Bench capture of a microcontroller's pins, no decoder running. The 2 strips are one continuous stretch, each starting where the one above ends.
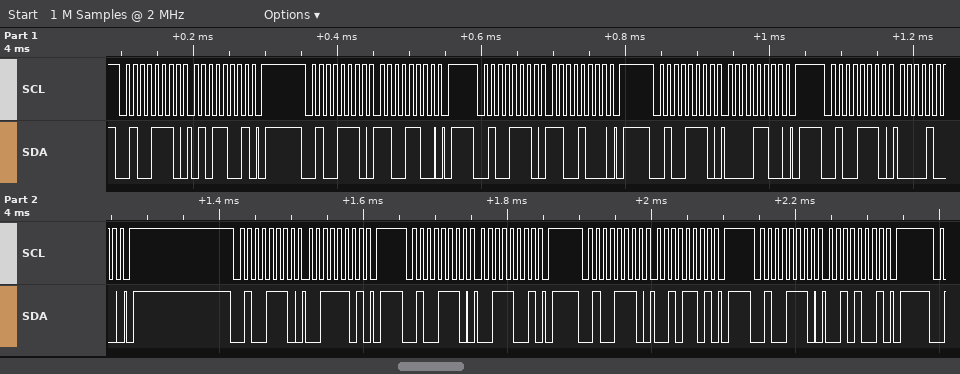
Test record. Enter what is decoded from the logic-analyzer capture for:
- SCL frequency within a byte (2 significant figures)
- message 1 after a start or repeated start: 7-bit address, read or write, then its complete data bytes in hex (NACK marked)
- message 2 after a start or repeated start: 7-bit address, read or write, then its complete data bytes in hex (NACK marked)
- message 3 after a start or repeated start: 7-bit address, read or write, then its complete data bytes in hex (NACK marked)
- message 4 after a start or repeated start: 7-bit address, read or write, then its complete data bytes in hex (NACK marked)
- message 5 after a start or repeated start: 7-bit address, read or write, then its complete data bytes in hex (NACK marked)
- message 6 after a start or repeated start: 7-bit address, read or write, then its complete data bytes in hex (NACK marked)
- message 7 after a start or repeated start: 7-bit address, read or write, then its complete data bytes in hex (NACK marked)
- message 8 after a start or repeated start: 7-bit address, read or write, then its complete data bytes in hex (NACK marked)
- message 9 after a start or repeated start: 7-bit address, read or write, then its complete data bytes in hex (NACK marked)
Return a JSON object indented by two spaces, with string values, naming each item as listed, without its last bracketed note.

{
  "SCL frequency within a byte": "100 kHz",
  "message 1 after a start or repeated start: 7-bit address, read or write, then its complete data bytes in hex": "0x27 write: 59",
  "message 2 after a start or repeated start: 7-bit address, read or write, then its complete data bytes in hex": "0x27 write: CC",
  "message 3 after a start or repeated start: 7-bit address, read or write, then its complete data bytes in hex": "0x27 write: C8",
  "message 4 after a start or repeated start: 7-bit address, read or write, then its complete data bytes in hex": "0x27 write: 0C",
  "message 5 after a start or repeated start: 7-bit address, read or write, then its complete data bytes in hex": "0x27 write: 08",
  "message 6 after a start or repeated start: 7-bit address, read or write, then its complete data bytes in hex": "0x27 write: 3D",
  "message 7 after a start or repeated start: 7-bit address, read or write, then its complete data bytes in hex": "0x27 write: 39",
  "message 8 after a start or repeated start: 7-bit address, read or write, then its complete data bytes in hex": "0x27 write: 2D",
  "message 9 after a start or repeated start: 7-bit address, read or write, then its complete data bytes in hex": "0x27 write: 29"
}
